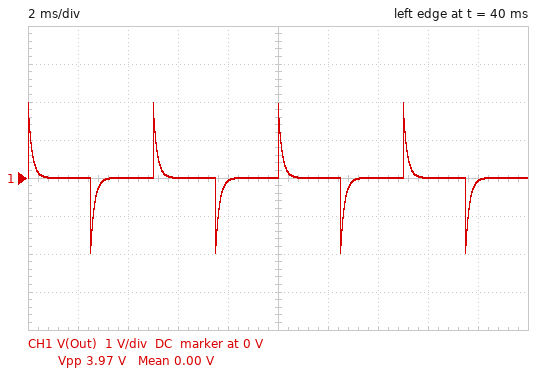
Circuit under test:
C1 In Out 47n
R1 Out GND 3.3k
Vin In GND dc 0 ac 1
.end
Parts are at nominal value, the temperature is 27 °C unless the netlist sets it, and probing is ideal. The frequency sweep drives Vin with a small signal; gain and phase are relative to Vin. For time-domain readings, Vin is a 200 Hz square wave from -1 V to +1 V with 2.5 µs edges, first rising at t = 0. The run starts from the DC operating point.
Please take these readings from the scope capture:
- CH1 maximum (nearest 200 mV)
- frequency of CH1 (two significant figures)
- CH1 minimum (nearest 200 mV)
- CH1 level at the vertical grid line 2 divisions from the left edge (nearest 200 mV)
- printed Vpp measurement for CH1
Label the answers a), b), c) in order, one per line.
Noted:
a) 2.0 V
b) 200 Hz
c) -2.0 V
d) 0 V
e) 3.97 V
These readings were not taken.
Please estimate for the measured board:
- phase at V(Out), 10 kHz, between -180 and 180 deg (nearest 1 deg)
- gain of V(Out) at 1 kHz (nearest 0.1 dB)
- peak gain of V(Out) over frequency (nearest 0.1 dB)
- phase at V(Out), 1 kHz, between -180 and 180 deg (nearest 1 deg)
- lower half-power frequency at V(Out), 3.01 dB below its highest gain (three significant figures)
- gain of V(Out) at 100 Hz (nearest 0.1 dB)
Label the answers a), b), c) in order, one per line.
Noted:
a) 6 deg
b) -3.1 dB
c) 0 dB
d) 46 deg
e) 1.03 kHz
f) -20.3 dB
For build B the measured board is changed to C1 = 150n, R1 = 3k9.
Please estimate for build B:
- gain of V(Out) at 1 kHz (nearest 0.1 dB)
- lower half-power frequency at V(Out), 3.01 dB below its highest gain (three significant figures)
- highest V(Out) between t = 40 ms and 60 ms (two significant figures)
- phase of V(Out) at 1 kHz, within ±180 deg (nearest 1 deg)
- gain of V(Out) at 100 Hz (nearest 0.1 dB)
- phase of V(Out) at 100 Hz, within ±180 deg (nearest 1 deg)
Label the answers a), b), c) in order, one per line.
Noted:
a) -0.3 dB
b) 272 Hz
c) 2.0 V
d) 15 deg
e) -9.2 dB
f) 70 deg
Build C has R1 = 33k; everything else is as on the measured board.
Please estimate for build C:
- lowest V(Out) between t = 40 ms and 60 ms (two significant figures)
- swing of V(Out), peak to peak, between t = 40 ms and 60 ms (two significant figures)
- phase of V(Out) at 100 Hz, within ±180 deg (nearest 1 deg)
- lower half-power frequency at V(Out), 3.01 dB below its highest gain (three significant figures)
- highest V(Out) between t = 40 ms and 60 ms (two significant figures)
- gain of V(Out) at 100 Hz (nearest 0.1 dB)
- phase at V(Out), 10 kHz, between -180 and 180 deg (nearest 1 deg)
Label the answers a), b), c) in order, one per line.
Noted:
a) -1.7 V
b) 3.3 V
c) 46 deg
d) 103 Hz
e) 1.7 V
f) -3.1 dB
g) 1 deg
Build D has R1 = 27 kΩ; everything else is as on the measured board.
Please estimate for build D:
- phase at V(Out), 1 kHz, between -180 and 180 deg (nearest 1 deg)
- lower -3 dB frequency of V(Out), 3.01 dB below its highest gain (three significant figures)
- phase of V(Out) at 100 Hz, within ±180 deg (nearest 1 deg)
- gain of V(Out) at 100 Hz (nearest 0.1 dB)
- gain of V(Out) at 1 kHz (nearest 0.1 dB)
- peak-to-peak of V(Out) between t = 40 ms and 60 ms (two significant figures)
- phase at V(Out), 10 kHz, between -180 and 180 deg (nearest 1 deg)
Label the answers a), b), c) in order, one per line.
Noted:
a) 7 deg
b) 125 Hz
c) 51 deg
d) -4.1 dB
e) -0.1 dB
f) 3.5 V
g) 1 deg
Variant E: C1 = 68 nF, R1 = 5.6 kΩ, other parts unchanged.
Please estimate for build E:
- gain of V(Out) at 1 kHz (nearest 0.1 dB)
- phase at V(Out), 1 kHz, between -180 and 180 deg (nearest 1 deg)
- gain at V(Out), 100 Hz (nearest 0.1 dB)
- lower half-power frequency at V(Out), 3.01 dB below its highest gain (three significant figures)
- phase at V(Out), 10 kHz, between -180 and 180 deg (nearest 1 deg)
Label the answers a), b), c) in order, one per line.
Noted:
a) -0.7 dB
b) 23 deg
c) -12.7 dB
d) 418 Hz
e) 2 deg
